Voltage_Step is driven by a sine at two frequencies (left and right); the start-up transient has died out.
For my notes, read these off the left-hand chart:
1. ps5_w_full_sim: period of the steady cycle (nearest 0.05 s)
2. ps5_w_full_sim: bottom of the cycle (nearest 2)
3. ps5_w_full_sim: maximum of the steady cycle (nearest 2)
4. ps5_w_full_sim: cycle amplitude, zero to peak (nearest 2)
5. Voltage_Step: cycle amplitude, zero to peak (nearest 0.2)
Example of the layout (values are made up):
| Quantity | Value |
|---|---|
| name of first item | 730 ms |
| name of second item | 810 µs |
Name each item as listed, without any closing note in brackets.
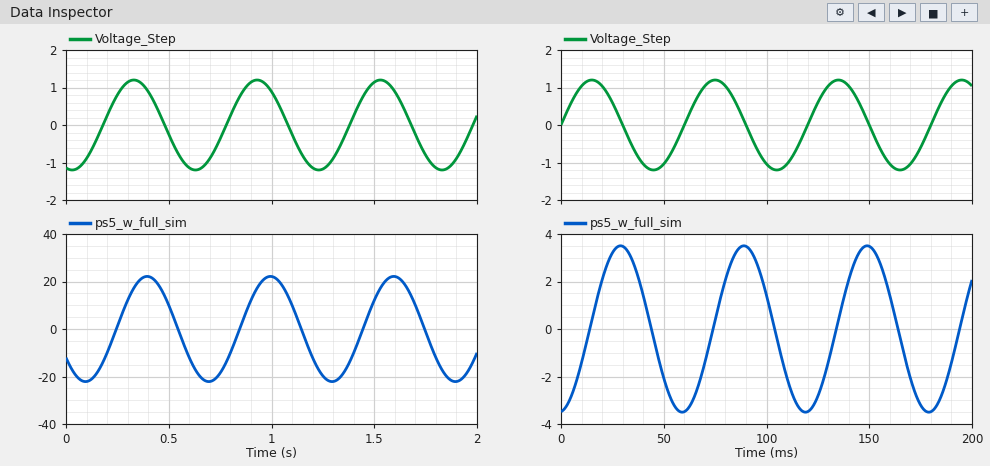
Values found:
| Quantity | Value |
|---|---|
| ps5_w_full_sim: period of the steady cycle | 0.60 s |
| ps5_w_full_sim: bottom of the cycle | -22 |
| ps5_w_full_sim: maximum of the steady cycle | 22 |
| ps5_w_full_sim: cycle amplitude, zero to peak | 22 |
| Voltage_Step: cycle amplitude, zero to peak | 1.2 |
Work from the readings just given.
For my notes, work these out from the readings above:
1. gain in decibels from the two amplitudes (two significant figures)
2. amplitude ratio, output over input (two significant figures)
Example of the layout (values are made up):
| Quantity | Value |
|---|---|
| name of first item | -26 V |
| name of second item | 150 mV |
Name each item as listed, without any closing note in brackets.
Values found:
| Quantity | Value |
|---|---|
| gain in decibels from the two amplitudes | 25 dB |
| amplitude ratio, output over input | 18 |
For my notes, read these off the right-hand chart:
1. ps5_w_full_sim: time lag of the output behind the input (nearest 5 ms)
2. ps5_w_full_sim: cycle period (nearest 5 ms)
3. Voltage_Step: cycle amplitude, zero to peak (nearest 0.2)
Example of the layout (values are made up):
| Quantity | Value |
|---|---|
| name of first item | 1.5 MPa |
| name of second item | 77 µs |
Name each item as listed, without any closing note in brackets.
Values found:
| Quantity | Value |
|---|---|
| ps5_w_full_sim: time lag of the output behind the input | 15 ms |
| ps5_w_full_sim: cycle period | 60 ms |
| Voltage_Step: cycle amplitude, zero to peak | 1.2 |
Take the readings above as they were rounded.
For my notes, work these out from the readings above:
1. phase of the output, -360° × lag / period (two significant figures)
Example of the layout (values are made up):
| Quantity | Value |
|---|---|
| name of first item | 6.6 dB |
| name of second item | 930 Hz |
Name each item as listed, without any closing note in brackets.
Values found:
| Quantity | Value |
|---|---|
| phase of the output, -360° × lag / period | -90° |
